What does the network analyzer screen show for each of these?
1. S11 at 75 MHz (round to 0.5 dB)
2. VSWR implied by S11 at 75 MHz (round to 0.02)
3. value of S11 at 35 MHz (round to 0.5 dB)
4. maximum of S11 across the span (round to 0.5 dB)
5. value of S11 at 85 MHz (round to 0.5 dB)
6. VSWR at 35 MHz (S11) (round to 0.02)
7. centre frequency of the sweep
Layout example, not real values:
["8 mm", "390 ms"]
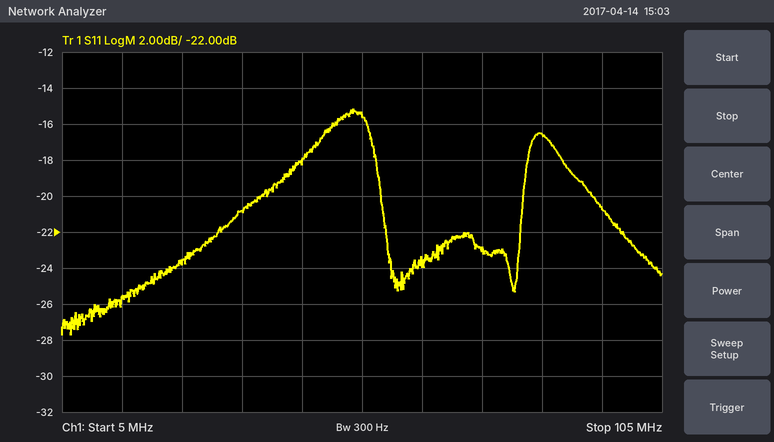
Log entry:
["-23.0 dB", "1.16", "-21.0 dB", "-15.0 dB", "-16.5 dB", "1.20", "55 MHz"]
